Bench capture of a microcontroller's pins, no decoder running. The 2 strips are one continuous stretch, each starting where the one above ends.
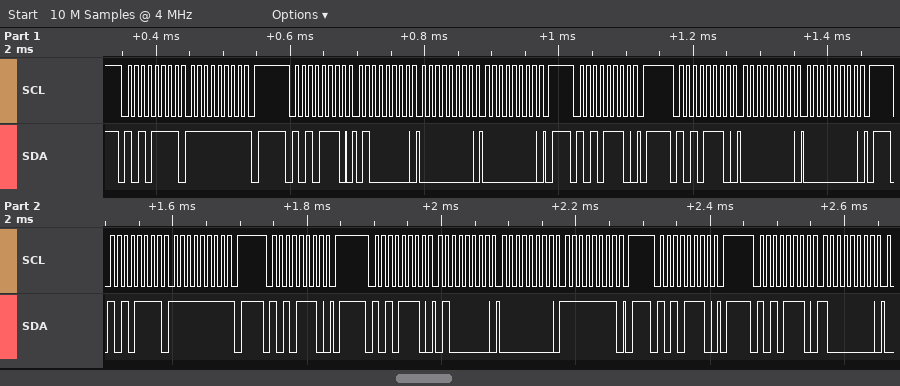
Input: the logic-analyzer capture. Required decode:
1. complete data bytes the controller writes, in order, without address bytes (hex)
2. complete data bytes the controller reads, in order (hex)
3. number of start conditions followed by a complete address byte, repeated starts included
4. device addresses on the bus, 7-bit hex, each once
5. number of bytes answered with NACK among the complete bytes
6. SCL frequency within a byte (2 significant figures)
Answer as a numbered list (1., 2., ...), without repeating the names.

1. 40 00 00 00 00 40 00 FF 80
2. FF FF
3. 9
4. 0x57
5. 2
6. 100 kHz
